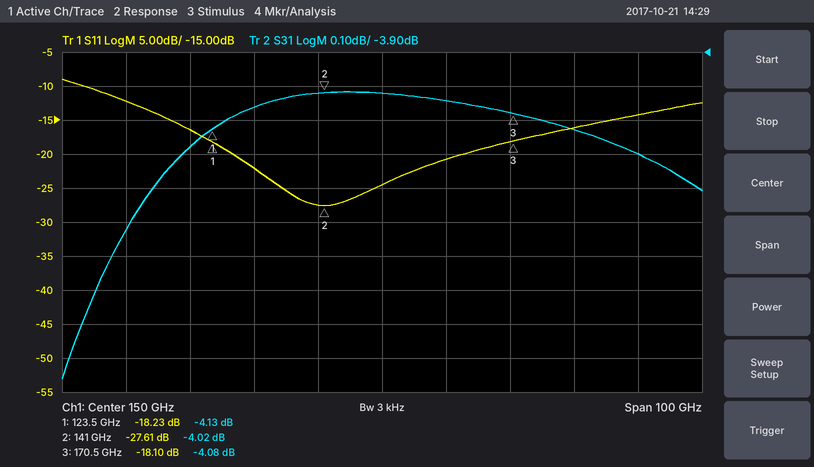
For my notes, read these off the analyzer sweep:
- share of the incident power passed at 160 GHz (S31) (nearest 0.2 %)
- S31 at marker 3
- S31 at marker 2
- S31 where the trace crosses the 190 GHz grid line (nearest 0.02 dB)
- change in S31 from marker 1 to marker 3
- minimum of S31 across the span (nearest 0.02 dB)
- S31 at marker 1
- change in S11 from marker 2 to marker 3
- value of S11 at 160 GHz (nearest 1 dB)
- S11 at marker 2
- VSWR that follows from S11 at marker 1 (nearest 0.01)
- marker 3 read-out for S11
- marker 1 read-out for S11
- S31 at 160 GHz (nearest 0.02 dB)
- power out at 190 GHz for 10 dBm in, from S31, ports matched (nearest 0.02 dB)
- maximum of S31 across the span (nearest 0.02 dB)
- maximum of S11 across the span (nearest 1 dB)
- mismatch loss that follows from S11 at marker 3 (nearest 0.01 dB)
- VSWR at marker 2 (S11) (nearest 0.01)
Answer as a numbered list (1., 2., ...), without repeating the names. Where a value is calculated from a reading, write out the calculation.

1. 10^(-4.04/10) ≈ 39.4 %
2. -4.08 dB
3. -4.02 dB
4. -4.20 dB
5. -4.08 − (-4.13) = 0.05 dB
6. -4.86 dB
7. -4.13 dB
8. -18.1 − (-27.61) = 9.51 dB
9. -21 dB
10. -27.61 dB
11. (1 + 0.1226)/(1 − 0.1226) ≈ 1.28
12. -18.10 dB
13. -18.23 dB
14. -4.04 dB
15. 10 dBm + (-4.20 dB) = 5.80 dBm
16. -4.02 dB
17. -9 dB
18. −10 log10(1 − 10^(-18.1/10)) ≈ 0.07 dB
19. (1 + 0.0416)/(1 − 0.0416) ≈ 1.09
